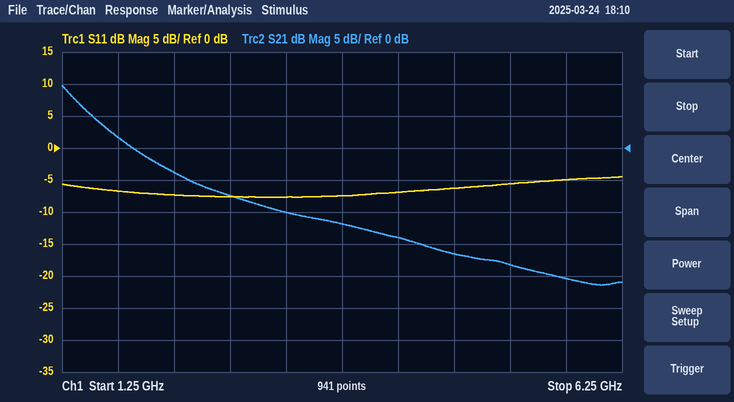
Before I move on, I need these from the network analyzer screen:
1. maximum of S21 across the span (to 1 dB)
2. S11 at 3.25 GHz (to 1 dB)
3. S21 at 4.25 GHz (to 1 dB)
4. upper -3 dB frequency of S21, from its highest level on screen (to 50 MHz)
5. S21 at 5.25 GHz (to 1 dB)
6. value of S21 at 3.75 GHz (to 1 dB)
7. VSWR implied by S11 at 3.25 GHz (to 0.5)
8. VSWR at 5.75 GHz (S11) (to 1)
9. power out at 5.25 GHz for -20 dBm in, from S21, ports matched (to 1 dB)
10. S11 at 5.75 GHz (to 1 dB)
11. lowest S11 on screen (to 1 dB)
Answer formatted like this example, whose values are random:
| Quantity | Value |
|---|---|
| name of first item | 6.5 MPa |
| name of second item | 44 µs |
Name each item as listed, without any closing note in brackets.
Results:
| Quantity | Value |
|---|---|
| maximum of S21 across the span | 10 dB |
| S11 at 3.25 GHz | -8 dB |
| S21 at 4.25 GHz | -14 dB |
| upper -3 dB frequency of S21, from its highest level on screen | 1.40 GHz |
| S21 at 5.25 GHz | -18 dB |
| value of S21 at 3.75 GHz | -12 dB |
| VSWR implied by S11 at 3.25 GHz | 2.5 |
| VSWR at 5.75 GHz (S11) | 4 |
| power out at 5.25 GHz for -20 dBm in, from S21, ports matched | -38 dBm |
| S11 at 5.75 GHz | -5 dB |
| lowest S11 on screen | -8 dB |
